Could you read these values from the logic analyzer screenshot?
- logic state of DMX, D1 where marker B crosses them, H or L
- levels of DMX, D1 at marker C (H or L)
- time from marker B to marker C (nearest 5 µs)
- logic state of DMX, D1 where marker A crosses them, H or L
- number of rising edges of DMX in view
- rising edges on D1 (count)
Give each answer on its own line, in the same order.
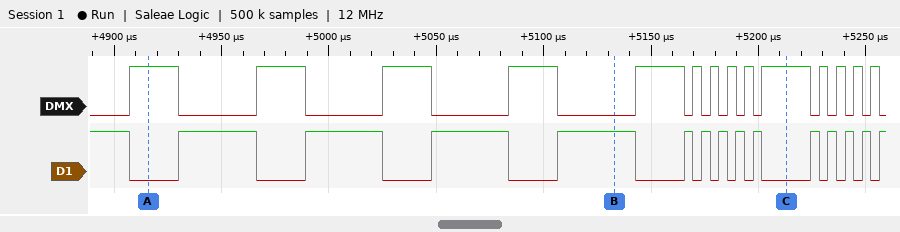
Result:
DMX=L, D1=H
DMX=H, D1=L
80 µs
DMX=H, D1=L
14
14
